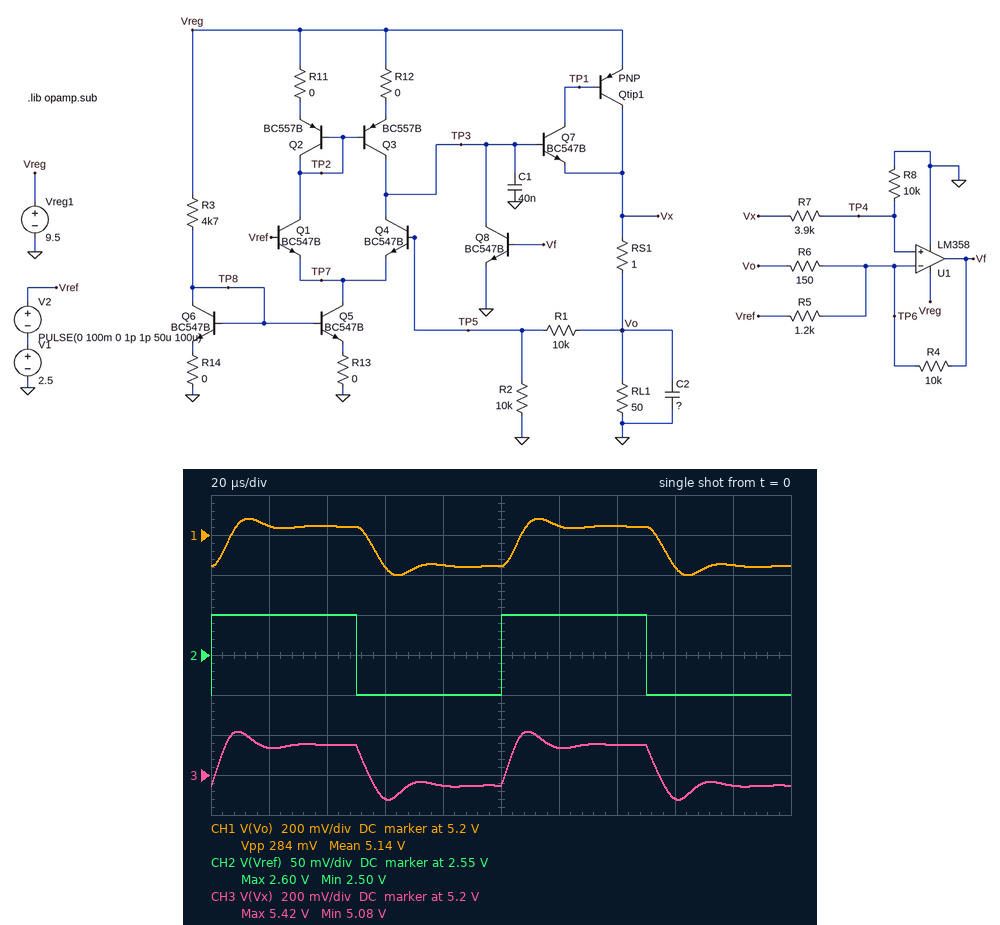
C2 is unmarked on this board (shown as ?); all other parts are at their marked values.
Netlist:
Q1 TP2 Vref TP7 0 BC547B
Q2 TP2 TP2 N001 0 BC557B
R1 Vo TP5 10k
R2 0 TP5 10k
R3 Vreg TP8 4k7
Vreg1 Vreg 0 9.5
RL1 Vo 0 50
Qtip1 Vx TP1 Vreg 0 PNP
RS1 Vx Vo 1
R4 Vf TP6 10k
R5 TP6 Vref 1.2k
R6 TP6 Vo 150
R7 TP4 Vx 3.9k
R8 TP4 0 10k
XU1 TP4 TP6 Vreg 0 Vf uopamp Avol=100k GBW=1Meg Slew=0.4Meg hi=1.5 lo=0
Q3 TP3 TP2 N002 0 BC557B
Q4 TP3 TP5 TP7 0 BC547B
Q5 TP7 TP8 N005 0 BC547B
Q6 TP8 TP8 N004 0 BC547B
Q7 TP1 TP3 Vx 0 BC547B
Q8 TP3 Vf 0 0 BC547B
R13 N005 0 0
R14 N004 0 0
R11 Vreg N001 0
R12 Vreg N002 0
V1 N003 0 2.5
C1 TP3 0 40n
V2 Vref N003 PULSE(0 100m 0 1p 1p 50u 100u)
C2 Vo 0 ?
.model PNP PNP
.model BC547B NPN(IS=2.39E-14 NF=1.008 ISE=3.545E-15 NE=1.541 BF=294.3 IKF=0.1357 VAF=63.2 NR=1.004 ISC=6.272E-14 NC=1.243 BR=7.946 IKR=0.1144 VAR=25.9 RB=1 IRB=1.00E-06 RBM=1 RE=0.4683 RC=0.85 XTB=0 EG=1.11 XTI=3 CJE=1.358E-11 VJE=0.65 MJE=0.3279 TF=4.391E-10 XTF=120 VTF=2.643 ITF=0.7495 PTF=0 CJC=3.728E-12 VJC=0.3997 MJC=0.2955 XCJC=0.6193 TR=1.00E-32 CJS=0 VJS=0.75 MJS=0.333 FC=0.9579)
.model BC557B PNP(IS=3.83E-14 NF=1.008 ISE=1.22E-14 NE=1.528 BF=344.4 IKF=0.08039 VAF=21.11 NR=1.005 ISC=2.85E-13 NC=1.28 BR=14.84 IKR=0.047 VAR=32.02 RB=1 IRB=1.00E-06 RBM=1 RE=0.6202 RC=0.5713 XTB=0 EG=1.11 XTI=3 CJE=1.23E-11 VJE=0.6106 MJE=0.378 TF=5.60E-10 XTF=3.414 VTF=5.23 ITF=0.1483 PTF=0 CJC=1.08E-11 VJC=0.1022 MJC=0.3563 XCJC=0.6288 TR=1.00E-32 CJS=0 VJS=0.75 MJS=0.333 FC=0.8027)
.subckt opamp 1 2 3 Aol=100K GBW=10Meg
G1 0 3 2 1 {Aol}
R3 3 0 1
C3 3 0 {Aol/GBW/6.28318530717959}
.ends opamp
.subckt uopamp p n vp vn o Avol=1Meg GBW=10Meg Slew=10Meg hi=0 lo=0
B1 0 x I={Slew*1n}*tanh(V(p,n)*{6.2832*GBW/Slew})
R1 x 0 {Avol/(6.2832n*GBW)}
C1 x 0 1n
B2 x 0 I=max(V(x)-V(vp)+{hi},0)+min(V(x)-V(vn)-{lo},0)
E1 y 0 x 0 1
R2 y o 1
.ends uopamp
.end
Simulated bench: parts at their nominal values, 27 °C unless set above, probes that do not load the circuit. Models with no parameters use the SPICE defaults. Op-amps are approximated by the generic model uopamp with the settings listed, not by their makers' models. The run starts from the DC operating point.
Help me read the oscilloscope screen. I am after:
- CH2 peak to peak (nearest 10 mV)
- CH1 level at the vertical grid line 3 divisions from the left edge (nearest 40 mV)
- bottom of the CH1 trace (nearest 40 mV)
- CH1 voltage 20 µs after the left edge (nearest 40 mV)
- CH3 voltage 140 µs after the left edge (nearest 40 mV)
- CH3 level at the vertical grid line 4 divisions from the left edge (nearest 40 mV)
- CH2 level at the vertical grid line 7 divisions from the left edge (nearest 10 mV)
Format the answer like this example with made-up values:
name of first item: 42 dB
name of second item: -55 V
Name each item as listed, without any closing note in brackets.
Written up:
CH2 peak to peak: 100 mV
CH1 level at the vertical grid line 3 divisions from the left edge: 5.04 V
bottom of the CH1 trace: 5.00 V
CH1 voltage 20 µs after the left edge: 5.24 V
CH3 voltage 140 µs after the left edge: 5.36 V
CH3 level at the vertical grid line 4 divisions from the left edge: 5.16 V
CH2 level at the vertical grid line 7 divisions from the left edge: 2.60 V
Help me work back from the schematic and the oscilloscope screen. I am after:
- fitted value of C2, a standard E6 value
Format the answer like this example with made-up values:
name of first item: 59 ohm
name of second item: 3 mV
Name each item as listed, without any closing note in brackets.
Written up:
fitted value of C2, a standard E6 value: 3.3 µF
